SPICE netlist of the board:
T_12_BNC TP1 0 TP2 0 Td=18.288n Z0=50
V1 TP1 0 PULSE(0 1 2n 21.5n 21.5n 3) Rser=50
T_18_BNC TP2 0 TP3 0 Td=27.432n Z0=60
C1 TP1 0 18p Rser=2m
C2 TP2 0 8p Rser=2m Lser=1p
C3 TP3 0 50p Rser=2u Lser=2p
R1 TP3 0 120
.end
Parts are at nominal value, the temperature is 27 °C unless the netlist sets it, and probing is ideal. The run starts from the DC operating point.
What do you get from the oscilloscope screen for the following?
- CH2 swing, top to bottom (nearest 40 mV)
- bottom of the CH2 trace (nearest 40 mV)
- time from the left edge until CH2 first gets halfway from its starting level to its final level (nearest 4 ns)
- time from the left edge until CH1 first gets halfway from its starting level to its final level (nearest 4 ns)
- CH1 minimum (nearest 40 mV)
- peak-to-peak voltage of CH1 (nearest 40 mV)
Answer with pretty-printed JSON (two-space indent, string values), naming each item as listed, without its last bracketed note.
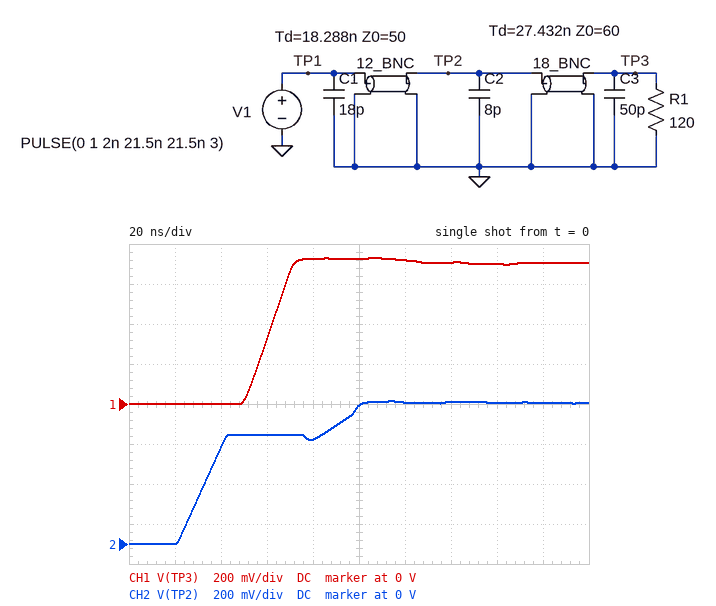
{
  "CH2 swing, top to bottom": "720 mV",
  "bottom of the CH2 trace": "0 V",
  "time from the left edge until CH2 first gets halfway from its starting level to its final level": "36 ns",
  "time from the left edge until CH1 first gets halfway from its starting level to its final level": "60 ns",
  "CH1 minimum": "0 V",
  "peak-to-peak voltage of CH1": "720 mV"
}
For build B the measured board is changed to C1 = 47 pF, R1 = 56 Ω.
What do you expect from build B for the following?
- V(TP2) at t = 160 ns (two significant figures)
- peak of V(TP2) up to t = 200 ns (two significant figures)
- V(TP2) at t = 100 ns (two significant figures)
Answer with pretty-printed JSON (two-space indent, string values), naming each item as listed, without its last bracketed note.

{
  "V(TP2) at t = 160 ns": "530 mV",
  "peak of V(TP2) up to t = 200 ns": "550 mV",
  "V(TP2) at t = 100 ns": "520 mV"
}
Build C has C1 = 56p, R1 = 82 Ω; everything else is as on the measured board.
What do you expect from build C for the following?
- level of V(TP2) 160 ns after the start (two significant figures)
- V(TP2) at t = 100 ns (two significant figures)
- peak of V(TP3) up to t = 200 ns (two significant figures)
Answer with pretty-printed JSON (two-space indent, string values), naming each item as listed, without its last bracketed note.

{
  "level of V(TP2) 160 ns after the start": "620 mV",
  "V(TP2) at t = 100 ns": "600 mV",
  "peak of V(TP3) up to t = 200 ns": "630 mV"
}
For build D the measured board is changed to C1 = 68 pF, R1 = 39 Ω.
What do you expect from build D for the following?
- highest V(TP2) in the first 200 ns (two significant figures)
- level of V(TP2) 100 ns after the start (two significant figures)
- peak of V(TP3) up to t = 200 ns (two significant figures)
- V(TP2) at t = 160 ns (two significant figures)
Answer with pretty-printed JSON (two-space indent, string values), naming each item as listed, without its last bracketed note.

{
  "highest V(TP2) in the first 200 ns": "550 mV",
  "level of V(TP2) 100 ns after the start": "430 mV",
  "peak of V(TP3) up to t = 200 ns": "450 mV",
  "V(TP2) at t = 160 ns": "440 mV"
}
